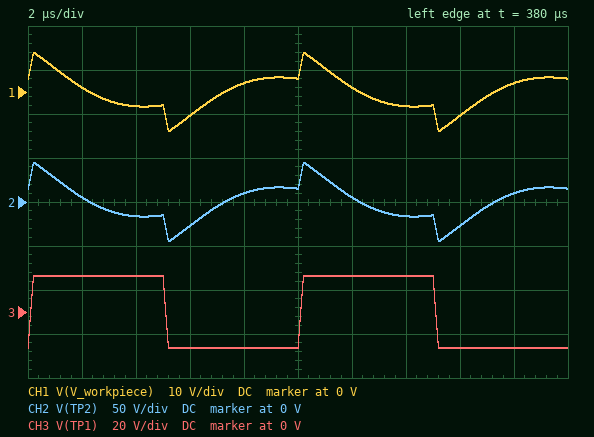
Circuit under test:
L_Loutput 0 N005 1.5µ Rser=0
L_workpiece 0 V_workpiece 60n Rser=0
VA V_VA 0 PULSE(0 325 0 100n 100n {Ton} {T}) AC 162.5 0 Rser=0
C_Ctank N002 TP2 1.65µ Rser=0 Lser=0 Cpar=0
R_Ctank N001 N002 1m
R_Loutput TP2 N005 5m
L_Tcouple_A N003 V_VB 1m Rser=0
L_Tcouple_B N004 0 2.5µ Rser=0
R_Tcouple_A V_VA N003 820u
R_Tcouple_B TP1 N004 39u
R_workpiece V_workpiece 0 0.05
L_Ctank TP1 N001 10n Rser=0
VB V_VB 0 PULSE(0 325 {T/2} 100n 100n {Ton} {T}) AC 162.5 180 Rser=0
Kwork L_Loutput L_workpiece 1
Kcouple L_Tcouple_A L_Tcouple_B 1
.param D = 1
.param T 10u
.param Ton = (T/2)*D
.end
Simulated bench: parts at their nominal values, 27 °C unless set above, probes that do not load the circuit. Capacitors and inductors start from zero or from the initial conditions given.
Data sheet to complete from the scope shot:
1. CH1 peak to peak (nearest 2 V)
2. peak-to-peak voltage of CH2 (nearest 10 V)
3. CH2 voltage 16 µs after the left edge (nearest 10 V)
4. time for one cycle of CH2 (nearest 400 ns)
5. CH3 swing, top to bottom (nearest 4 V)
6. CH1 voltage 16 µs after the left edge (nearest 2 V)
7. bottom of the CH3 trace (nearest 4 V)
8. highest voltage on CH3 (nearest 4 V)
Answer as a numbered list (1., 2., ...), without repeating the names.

1. 18 V
2. 90 V
3. -30 V
4. 10.0 µs
5. 32 V
6. -6 V
7. -16 V
8. 16 V
